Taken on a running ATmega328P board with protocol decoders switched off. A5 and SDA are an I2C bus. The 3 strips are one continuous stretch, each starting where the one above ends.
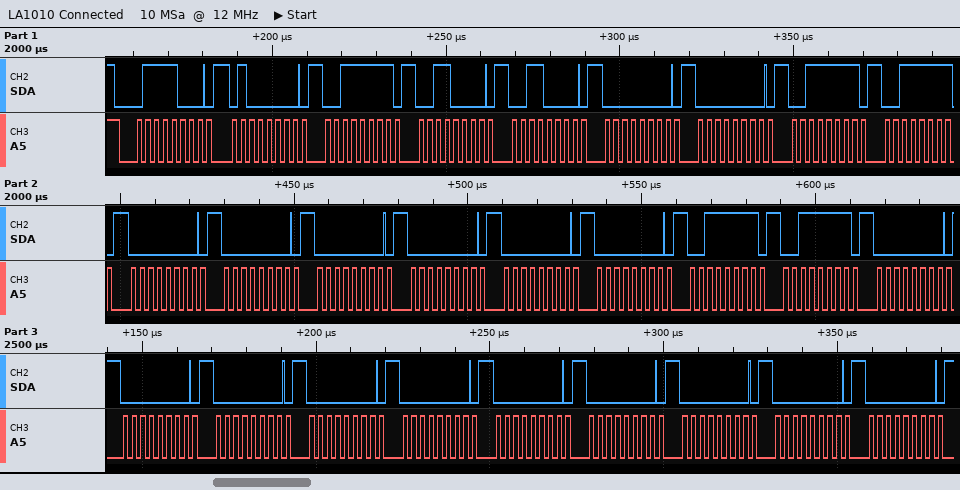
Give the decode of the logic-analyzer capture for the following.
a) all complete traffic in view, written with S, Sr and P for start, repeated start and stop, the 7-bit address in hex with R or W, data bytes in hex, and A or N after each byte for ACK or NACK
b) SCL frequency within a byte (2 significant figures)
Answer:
S 3CW A 40 A 3F A 30 A 30 A 00 A 00 A 3F A 3F A 00 A 00 A 00 A 00 A 00 A 00 A 3F A 3F A 00 A 00 A 00 A 00 A 00 A 00 A 00 A 00 A 00 A 00 A
400 kHz
